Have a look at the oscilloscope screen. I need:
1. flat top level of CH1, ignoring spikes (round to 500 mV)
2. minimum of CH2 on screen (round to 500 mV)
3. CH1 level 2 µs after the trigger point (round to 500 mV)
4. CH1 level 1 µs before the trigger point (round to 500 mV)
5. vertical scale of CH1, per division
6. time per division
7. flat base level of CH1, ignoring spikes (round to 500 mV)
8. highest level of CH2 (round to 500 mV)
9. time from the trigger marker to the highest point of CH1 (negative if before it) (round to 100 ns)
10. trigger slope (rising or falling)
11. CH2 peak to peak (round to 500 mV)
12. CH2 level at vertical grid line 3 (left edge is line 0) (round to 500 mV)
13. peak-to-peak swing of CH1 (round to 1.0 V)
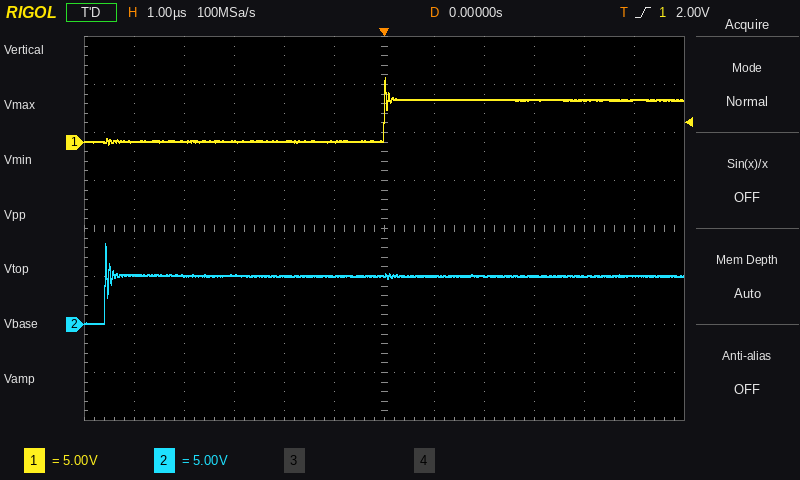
4.5 V
0.0 V
4.5 V
0.0 V
5 V
1 µs
0.0 V
8.5 V
0.0 µs
rising
8.5 V
5.0 V
7.0 V
